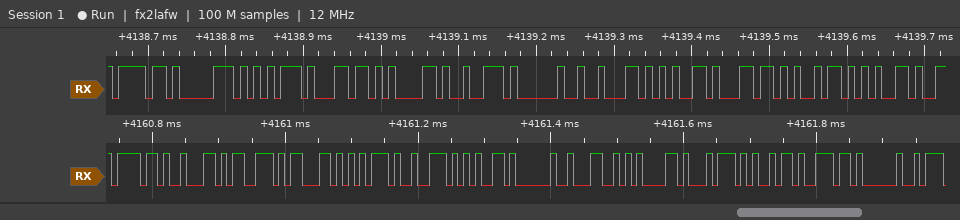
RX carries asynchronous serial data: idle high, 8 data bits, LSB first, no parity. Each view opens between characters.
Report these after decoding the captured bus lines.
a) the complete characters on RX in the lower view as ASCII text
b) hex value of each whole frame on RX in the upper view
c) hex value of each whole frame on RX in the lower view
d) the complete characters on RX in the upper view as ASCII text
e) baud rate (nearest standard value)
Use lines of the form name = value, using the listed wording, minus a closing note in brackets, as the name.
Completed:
the complete characters on RX in the lower view as ASCII text = "obscure Latin "
hex value of each whole frame on RX in the upper view = 6F, 70, 75, 6C, 61, 72, 20, 62, 65, 6C, 69, 65
hex value of each whole frame on RX in the lower view = 6F, 62, 73, 63, 75, 72, 65, 20, 4C, 61, 74, 69, 6E, 20
the complete characters on RX in the upper view as ASCII text = "opular belie"
baud rate = 115200 baud
